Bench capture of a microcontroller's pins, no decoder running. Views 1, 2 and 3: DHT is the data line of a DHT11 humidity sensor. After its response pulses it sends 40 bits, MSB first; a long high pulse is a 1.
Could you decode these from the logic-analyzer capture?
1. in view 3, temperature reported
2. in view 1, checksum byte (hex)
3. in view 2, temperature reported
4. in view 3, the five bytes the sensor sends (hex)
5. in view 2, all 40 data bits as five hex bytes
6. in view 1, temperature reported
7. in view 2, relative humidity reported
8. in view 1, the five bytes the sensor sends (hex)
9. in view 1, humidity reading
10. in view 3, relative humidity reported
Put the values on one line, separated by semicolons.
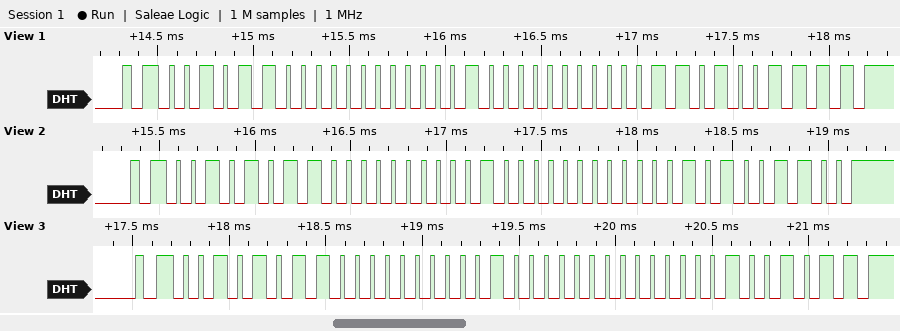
32.0 °C; 0x4F; 32.1 °C; 2B 00 20 00 4B; 2B 00 20 01 4C; 32.3 °C; 43 %; 2C 00 20 03 4F; 44 %; 43 %
